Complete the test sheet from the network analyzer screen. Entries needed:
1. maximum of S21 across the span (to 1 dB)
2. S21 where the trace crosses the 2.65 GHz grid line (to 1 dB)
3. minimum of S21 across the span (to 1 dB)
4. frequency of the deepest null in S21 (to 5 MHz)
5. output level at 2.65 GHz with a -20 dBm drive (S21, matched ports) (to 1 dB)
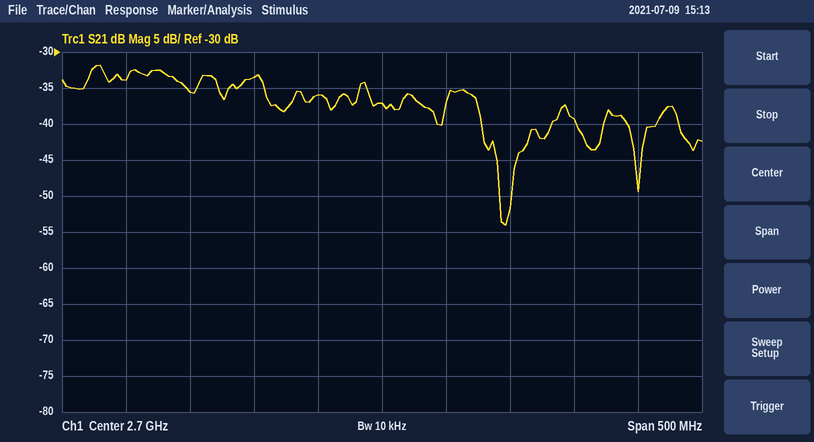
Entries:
-32 dB
-36 dB
-54 dB
2.795 GHz
-56 dBm
